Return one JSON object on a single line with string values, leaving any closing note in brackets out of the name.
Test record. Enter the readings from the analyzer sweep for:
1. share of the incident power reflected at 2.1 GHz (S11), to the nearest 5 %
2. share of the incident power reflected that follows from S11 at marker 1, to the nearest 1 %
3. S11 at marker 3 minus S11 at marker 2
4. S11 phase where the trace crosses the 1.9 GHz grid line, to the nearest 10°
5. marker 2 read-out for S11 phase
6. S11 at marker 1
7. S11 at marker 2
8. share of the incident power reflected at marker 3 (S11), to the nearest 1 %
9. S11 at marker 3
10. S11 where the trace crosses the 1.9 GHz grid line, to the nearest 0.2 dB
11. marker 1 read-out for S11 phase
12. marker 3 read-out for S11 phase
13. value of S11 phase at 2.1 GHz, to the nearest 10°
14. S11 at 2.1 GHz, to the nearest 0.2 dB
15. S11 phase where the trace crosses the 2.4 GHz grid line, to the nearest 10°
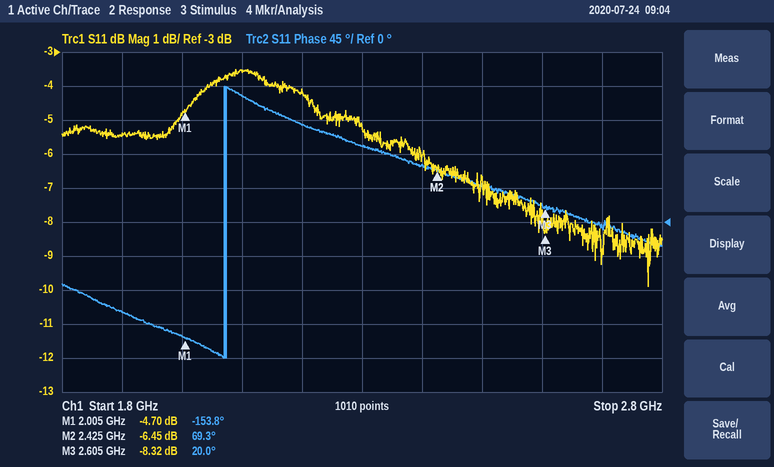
{"share of the incident power reflected at 2.1 GHz (S11), to the nearest 5 %": "45 %", "share of the incident power reflected that follows from S11 at marker 1, to the nearest 1 %": "34 %", "S11 at marker 3 minus S11 at marker 2": "-1.87 dB", "S11 phase where the trace crosses the 1.9 GHz grid line, to the nearest 10°": "-120°", "marker 2 read-out for S11 phase": "69.3°", "S11 at marker 1": "-4.70 dB", "S11 at marker 2": "-6.45 dB", "share of the incident power reflected at marker 3 (S11), to the nearest 1 %": "15 %", "S11 at marker 3": "-8.32 dB", "S11 where the trace crosses the 1.9 GHz grid line, to the nearest 0.2 dB": "-5.4 dB", "marker 1 read-out for S11 phase": "-153.8°", "marker 3 read-out for S11 phase": "20.0°", "value of S11 phase at 2.1 GHz, to the nearest 10°": "170°", "S11 at 2.1 GHz, to the nearest 0.2 dB": "-3.6 dB", "S11 phase where the trace crosses the 2.4 GHz grid line, to the nearest 10°": "80°"}
